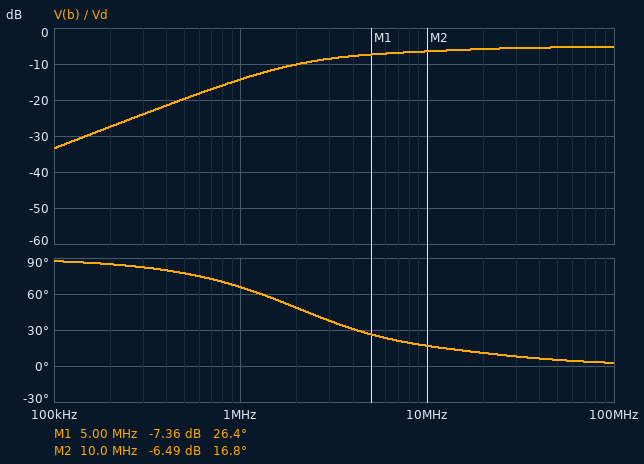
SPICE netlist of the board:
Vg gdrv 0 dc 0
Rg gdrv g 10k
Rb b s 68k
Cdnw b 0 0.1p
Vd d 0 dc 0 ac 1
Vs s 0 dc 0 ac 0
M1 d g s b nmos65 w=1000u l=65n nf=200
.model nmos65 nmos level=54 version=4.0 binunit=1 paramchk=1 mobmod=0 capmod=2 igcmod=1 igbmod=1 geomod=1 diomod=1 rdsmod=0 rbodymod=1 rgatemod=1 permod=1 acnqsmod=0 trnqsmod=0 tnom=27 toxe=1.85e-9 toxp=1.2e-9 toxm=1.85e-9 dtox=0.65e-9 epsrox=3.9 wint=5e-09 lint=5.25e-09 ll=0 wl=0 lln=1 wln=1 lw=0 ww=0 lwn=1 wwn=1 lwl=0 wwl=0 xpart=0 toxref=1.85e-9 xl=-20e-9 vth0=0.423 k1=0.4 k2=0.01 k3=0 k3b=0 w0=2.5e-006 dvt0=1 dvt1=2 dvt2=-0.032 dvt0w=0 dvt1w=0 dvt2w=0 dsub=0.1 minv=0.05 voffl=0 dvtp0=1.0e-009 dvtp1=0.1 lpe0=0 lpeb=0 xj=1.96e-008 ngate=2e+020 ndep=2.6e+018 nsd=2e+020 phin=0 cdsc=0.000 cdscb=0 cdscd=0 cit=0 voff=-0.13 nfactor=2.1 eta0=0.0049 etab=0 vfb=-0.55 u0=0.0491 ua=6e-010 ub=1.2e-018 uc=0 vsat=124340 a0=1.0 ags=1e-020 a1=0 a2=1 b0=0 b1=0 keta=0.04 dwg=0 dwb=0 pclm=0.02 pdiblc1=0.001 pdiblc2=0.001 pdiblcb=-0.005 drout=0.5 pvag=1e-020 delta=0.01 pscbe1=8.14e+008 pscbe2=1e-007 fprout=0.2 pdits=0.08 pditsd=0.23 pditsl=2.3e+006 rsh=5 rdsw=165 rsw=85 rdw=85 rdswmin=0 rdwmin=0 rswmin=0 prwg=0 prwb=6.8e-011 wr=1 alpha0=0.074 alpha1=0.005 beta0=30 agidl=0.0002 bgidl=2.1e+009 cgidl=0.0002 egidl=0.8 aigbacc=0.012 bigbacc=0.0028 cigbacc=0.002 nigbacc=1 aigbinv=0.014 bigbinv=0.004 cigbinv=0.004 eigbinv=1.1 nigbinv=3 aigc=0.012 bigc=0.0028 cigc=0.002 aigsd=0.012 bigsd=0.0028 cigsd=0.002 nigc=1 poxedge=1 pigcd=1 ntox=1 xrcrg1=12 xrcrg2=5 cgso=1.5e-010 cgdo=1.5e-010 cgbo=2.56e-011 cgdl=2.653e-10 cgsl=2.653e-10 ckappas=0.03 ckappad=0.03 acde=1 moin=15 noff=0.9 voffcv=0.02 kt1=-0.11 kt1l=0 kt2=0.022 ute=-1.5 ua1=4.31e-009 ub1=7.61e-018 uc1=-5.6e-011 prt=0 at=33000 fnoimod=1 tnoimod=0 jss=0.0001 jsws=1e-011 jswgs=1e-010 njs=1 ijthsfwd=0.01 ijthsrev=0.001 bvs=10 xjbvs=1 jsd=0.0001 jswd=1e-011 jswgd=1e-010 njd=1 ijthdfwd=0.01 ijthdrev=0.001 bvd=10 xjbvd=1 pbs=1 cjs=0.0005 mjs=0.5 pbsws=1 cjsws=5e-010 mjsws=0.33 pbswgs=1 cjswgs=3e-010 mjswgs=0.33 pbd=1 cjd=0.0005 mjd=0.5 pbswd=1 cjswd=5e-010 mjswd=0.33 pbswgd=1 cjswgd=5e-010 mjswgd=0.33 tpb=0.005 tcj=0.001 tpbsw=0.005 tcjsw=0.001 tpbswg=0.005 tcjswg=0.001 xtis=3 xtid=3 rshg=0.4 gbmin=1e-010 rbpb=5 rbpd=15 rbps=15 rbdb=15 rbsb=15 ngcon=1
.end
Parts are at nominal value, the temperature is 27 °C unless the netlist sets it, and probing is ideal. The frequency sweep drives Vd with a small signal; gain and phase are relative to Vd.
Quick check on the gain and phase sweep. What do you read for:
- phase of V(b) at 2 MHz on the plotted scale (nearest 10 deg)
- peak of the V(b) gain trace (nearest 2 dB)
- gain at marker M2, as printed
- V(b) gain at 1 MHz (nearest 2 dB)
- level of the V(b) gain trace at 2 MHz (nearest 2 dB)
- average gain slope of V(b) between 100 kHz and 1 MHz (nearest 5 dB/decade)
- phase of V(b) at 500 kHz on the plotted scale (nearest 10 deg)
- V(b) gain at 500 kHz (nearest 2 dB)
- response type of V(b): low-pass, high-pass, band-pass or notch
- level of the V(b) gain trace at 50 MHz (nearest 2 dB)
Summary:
50 deg
-6 dB
-6.49 dB
-14 dB
-10 dB
20 dB/decade
80 deg
-20 dB
high-pass
-6 dB
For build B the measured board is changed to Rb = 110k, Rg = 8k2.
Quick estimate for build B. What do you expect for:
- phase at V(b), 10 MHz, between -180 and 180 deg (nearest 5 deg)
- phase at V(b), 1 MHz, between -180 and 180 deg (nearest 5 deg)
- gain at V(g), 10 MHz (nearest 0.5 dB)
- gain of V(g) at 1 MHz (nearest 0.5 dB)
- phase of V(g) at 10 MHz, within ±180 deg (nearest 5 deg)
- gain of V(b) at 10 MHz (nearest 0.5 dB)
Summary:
10 deg
55 deg
-12.5 dB
-32.5 dB
65 deg
-6.5 dB
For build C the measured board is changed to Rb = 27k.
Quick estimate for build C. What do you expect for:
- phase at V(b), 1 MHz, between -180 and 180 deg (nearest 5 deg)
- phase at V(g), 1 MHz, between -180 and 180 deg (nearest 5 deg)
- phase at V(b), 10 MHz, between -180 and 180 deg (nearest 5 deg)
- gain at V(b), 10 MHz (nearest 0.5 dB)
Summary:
80 deg
90 deg
35 deg
-7.5 dB
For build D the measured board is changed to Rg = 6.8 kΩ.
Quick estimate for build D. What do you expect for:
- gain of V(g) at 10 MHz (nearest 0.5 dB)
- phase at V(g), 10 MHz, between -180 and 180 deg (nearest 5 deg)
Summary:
-14.0 dB
70 deg
